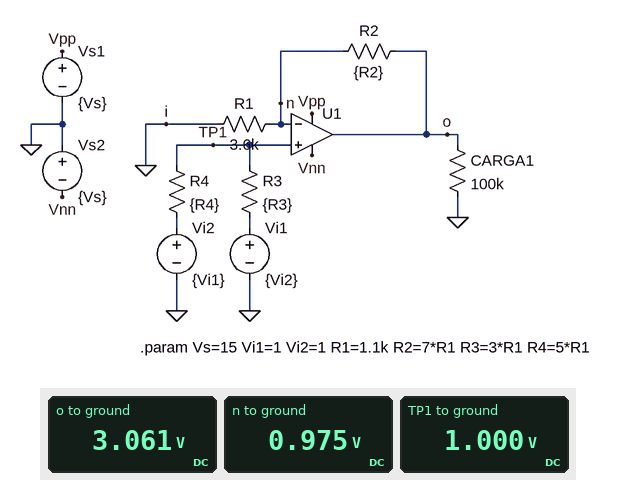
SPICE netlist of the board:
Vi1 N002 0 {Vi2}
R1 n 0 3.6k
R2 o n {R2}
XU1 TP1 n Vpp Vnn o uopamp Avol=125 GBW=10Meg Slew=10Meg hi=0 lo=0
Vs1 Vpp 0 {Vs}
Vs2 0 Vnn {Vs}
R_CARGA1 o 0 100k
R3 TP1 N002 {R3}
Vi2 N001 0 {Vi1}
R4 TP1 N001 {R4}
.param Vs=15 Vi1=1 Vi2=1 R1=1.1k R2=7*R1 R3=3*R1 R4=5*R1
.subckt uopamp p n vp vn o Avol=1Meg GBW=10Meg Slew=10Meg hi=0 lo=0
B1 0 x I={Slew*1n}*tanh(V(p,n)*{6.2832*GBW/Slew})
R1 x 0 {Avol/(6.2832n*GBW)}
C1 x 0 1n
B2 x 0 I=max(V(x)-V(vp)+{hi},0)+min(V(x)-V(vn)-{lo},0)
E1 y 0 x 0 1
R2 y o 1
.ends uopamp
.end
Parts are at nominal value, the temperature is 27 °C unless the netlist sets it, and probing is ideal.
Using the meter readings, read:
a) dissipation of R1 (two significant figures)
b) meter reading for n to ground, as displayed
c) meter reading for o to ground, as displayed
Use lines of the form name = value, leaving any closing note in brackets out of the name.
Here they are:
dissipation of R1 = 260 µW
meter reading for n to ground, as displayed = 0.975 V
meter reading for o to ground, as displayed = 3.061 V
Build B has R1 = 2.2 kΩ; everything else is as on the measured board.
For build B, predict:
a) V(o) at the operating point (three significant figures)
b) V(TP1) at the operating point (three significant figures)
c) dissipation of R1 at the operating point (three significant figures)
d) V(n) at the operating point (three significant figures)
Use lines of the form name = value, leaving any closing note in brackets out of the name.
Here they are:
V(o) at the operating point = 4.34 V
V(TP1) at the operating point = 1.00 V
dissipation of R1 at the operating point = 423 µW
V(n) at the operating point = 965 mV
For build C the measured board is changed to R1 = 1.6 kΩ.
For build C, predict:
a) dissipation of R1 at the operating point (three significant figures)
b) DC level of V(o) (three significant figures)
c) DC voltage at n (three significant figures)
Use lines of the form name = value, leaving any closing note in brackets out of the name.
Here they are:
dissipation of R1 at the operating point = 569 µW
DC level of V(o) = 5.55 V
DC voltage at n = 954 mV
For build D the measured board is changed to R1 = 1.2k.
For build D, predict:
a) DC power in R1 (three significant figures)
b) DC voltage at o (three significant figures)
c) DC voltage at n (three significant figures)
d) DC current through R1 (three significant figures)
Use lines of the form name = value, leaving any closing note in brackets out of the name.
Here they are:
DC power in R1 = 739 µW
DC voltage at o = 6.98 V
DC voltage at n = 942 mV
DC current through R1 = 785 µA
